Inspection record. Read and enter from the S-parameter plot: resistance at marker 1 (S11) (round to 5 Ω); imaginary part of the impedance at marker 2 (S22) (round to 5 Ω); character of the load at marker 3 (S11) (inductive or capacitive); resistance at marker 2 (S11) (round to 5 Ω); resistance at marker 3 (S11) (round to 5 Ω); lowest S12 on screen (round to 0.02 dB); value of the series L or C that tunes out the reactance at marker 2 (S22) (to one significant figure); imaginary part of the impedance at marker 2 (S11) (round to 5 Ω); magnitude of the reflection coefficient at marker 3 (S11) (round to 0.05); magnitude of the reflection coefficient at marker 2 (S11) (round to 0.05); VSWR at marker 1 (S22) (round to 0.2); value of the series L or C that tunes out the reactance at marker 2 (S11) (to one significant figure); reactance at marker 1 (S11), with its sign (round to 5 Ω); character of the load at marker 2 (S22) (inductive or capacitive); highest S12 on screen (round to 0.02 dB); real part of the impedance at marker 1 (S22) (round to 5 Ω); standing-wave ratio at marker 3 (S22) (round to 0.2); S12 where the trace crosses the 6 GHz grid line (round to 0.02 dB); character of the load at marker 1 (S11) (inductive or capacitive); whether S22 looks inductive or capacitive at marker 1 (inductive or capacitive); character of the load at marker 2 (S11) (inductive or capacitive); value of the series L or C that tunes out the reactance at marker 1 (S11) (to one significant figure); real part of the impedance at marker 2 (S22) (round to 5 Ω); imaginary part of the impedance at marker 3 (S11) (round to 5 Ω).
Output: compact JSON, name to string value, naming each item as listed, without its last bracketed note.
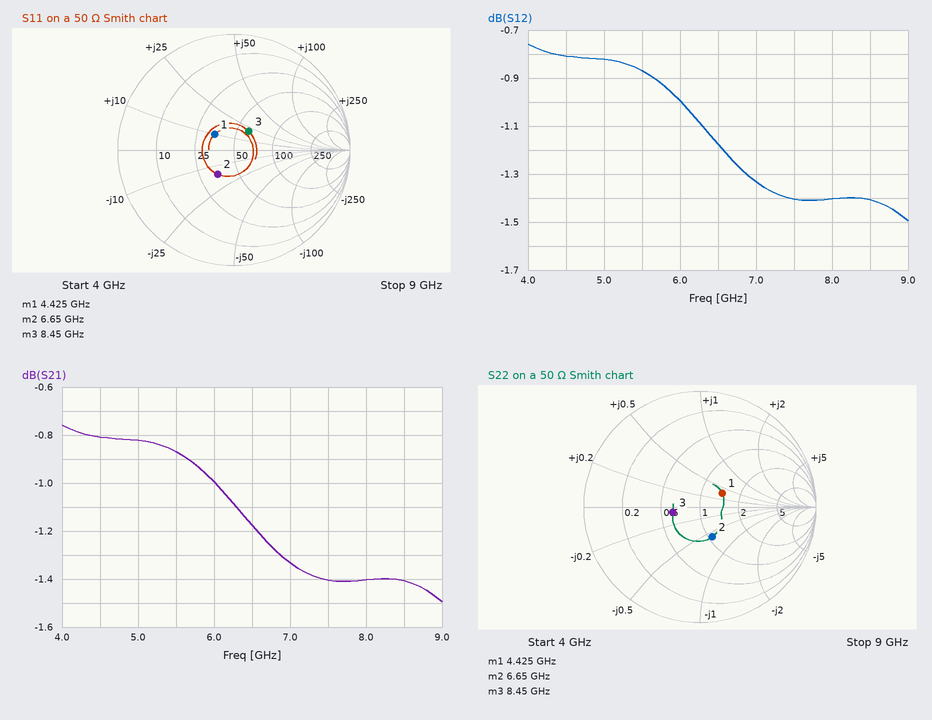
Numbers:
{"resistance at marker 1 (S11)": "35 Ω", "imaginary part of the impedance at marker 2 (S22)": "-30 Ω", "character of the load at marker 3 (S11)": "inductive", "resistance at marker 2 (S11)": "35 Ω", "resistance at marker 3 (S11)": "60 Ω", "lowest S12 on screen": "-1.50 dB", "value of the series L or C that tunes out the reactance at marker 2 (S22)": "700 pH", "imaginary part of the impedance at marker 2 (S11)": "-15 Ω", "magnitude of the reflection coefficient at marker 3 (S11)": "0.20", "magnitude of the reflection coefficient at marker 2 (S11)": "0.25", "VSWR at marker 1 (S22)": "1.6", "value of the series L or C that tunes out the reactance at marker 2 (S11)": "400 pH", "reactance at marker 1 (S11), with its sign": "+10 Ω", "character of the load at marker 2 (S22)": "capacitive", "highest S12 on screen": "-0.76 dB", "real part of the impedance at marker 1 (S22)": "70 Ω", "standing-wave ratio at marker 3 (S22)": "1.6", "S12 where the trace crosses the 6 GHz grid line": "-1.00 dB", "character of the load at marker 1 (S11)": "inductive", "whether S22 looks inductive or capacitive at marker 1": "inductive", "character of the load at marker 2 (S11)": "capacitive", "value of the series L or C that tunes out the reactance at marker 1 (S11)": "4 pF", "real part of the impedance at marker 2 (S22)": "55 Ω", "imaginary part of the impedance at marker 3 (S11)": "+20 Ω"}
